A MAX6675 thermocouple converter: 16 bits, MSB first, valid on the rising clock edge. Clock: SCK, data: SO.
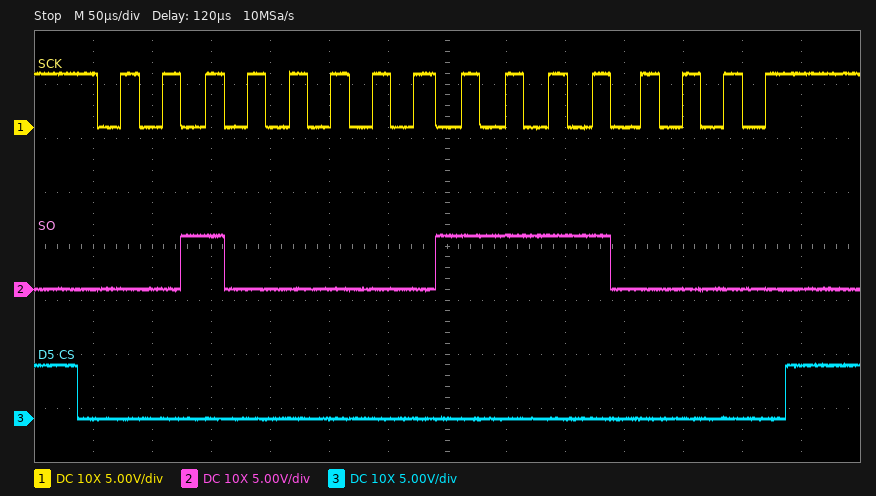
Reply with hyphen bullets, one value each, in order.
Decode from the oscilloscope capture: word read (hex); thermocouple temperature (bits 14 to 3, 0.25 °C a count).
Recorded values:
- 0x20F0
- 263.50 °C
